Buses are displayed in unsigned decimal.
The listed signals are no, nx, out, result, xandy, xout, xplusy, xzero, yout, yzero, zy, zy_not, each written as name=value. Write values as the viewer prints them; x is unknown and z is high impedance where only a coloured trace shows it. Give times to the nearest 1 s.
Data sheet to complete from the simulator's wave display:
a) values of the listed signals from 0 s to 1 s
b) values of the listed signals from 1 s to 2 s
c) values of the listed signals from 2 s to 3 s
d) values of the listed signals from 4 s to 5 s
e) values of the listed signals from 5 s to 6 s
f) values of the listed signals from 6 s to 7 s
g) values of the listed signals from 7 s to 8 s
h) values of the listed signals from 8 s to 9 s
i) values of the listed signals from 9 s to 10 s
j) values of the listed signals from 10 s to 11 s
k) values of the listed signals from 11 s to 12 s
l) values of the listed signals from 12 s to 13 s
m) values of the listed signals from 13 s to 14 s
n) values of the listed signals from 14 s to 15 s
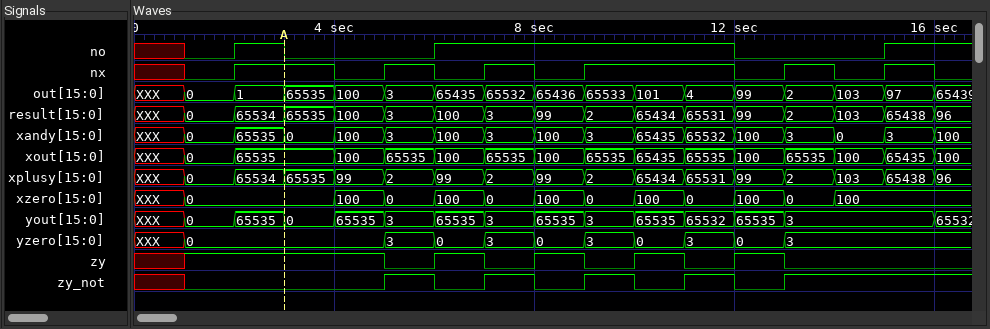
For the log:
no=x, nx=x, out=XXX, result=XXX, xandy=XXX, xout=XXX, xplusy=XXX, xzero=XXX, yout=XXX, yzero=XXX, zy=x, zy_not=x
no=0, nx=0, out=0, result=0, xandy=0, xout=0, xplusy=0, xzero=0, yout=0, yzero=0, zy=1, zy_not=0
no=1, nx=1, out=1, result=65534, xandy=65535, xout=65535, xplusy=65534, xzero=0, yout=65535, yzero=0, zy=1, zy_not=0
no=0, nx=0, out=100, result=100, xandy=100, xout=100, xplusy=99, xzero=100, yout=65535, yzero=0, zy=1, zy_not=0
no=0, nx=1, out=3, result=3, xandy=3, xout=65535, xplusy=2, xzero=0, yout=3, yzero=3, zy=0, zy_not=1
no=1, nx=0, out=65435, result=100, xandy=100, xout=100, xplusy=99, xzero=100, yout=65535, yzero=0, zy=1, zy_not=0
no=1, nx=1, out=65532, result=3, xandy=3, xout=65535, xplusy=2, xzero=0, yout=3, yzero=3, zy=0, zy_not=1
no=1, nx=0, out=65436, result=99, xandy=100, xout=100, xplusy=99, xzero=100, yout=65535, yzero=0, zy=1, zy_not=0
no=1, nx=1, out=65533, result=2, xandy=3, xout=65535, xplusy=2, xzero=0, yout=3, yzero=3, zy=0, zy_not=1
no=1, nx=1, out=101, result=65434, xandy=65435, xout=65435, xplusy=65434, xzero=100, yout=65535, yzero=0, zy=1, zy_not=0
no=1, nx=1, out=4, result=65531, xandy=65532, xout=65535, xplusy=65531, xzero=0, yout=65532, yzero=3, zy=0, zy_not=1
no=0, nx=0, out=99, result=99, xandy=100, xout=100, xplusy=99, xzero=100, yout=65535, yzero=0, zy=1, zy_not=0
no=0, nx=1, out=2, result=2, xandy=3, xout=65535, xplusy=2, xzero=0, yout=3, yzero=3, zy=0, zy_not=1
no=0, nx=0, out=103, result=103, xandy=0, xout=100, xplusy=103, xzero=100, yout=3, yzero=3, zy=0, zy_not=1
